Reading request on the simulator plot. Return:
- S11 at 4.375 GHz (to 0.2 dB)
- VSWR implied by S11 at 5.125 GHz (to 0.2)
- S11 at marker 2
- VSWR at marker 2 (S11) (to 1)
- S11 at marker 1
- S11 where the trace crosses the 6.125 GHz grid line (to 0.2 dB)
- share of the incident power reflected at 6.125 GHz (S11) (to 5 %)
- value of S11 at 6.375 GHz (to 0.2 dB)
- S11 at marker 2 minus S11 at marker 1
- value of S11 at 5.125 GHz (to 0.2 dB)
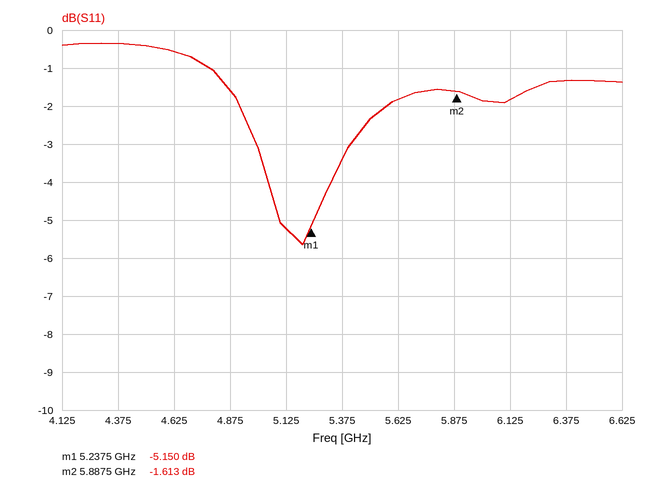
-0.4 dB
3.4
-1.613 dB
11
-5.150 dB
-1.8 dB
65 %
-1.4 dB
3.537 dB
-5.2 dB
